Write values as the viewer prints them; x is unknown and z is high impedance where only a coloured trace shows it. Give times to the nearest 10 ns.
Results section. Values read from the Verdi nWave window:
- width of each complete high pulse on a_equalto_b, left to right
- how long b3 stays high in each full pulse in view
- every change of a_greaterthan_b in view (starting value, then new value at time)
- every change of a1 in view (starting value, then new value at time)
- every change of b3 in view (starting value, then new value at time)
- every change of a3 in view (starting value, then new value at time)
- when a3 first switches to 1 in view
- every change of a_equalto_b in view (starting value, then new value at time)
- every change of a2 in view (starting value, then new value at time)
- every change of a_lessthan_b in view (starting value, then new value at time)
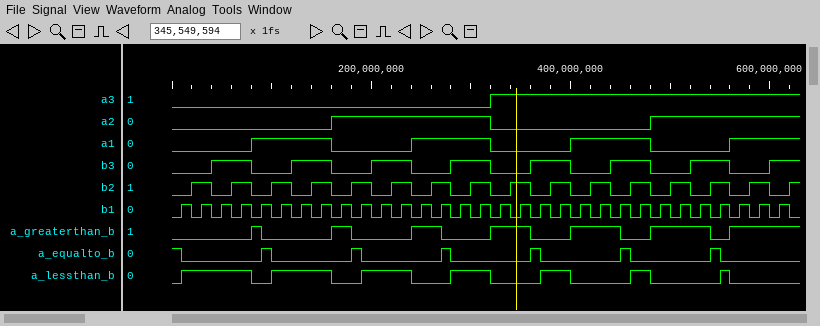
10 ns, 10 ns, 10 ns, 10 ns, 10 ns, 10 ns
40 ns, 40 ns, 40 ns, 40 ns, 40 ns, 40 ns, 40 ns
0, 1 at 80 ns, 0 at 90 ns, 1 at 160 ns, 0 at 180 ns, 1 at 240 ns, 0 at 270 ns, 1 at 320 ns, 0 at 360 ns, 1 at 400 ns, 0 at 450 ns, 1 at 480 ns, 0 at 540 ns, 1 at 560 ns
0, 1 at 80 ns, 0 at 160 ns, 1 at 240 ns, 0 at 320 ns, 1 at 400 ns, 0 at 480 ns, 1 at 560 ns
0, 1 at 40 ns, 0 at 80 ns, 1 at 120 ns, 0 at 160 ns, 1 at 200 ns, 0 at 240 ns, 1 at 280 ns, 0 at 320 ns, 1 at 360 ns, 0 at 400 ns, 1 at 440 ns, 0 at 480 ns, 1 at 520 ns, 0 at 560 ns, 1 at 600 ns
0, 1 at 320 ns
320 ns
1, 0 at 10 ns, 1 at 90 ns, 0 at 100 ns, 1 at 180 ns, 0 at 190 ns, 1 at 270 ns, 0 at 280 ns, 1 at 360 ns, 0 at 370 ns, 1 at 450 ns, 0 at 460 ns, 1 at 540 ns, 0 at 550 ns
0, 1 at 160 ns, 0 at 320 ns, 1 at 480 ns
0, 1 at 10 ns, 0 at 80 ns, 1 at 100 ns, 0 at 160 ns, 1 at 190 ns, 0 at 240 ns, 1 at 280 ns, 0 at 320 ns, 1 at 370 ns, 0 at 400 ns, 1 at 460 ns, 0 at 480 ns, 1 at 550 ns, 0 at 560 ns
